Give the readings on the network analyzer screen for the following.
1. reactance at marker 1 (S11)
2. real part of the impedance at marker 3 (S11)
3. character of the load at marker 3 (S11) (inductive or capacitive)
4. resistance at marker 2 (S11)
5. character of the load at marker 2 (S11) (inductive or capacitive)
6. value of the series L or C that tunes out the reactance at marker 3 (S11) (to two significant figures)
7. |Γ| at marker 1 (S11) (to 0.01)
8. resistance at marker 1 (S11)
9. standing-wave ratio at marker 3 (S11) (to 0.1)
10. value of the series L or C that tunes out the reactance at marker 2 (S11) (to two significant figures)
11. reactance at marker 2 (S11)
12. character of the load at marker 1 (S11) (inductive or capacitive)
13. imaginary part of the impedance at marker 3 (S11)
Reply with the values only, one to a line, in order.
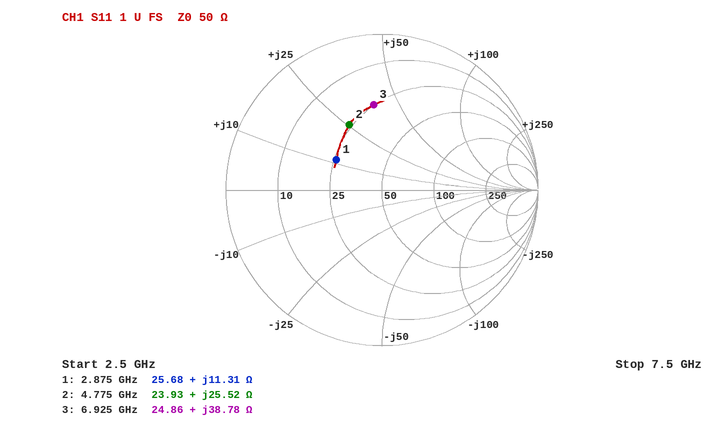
+11.31 Ω
24.86 Ω
inductive
23.93 Ω
inductive
590 fF
0.35
25.68 Ω
3.4
1.3 pF
+25.52 Ω
inductive
+38.78 Ω
